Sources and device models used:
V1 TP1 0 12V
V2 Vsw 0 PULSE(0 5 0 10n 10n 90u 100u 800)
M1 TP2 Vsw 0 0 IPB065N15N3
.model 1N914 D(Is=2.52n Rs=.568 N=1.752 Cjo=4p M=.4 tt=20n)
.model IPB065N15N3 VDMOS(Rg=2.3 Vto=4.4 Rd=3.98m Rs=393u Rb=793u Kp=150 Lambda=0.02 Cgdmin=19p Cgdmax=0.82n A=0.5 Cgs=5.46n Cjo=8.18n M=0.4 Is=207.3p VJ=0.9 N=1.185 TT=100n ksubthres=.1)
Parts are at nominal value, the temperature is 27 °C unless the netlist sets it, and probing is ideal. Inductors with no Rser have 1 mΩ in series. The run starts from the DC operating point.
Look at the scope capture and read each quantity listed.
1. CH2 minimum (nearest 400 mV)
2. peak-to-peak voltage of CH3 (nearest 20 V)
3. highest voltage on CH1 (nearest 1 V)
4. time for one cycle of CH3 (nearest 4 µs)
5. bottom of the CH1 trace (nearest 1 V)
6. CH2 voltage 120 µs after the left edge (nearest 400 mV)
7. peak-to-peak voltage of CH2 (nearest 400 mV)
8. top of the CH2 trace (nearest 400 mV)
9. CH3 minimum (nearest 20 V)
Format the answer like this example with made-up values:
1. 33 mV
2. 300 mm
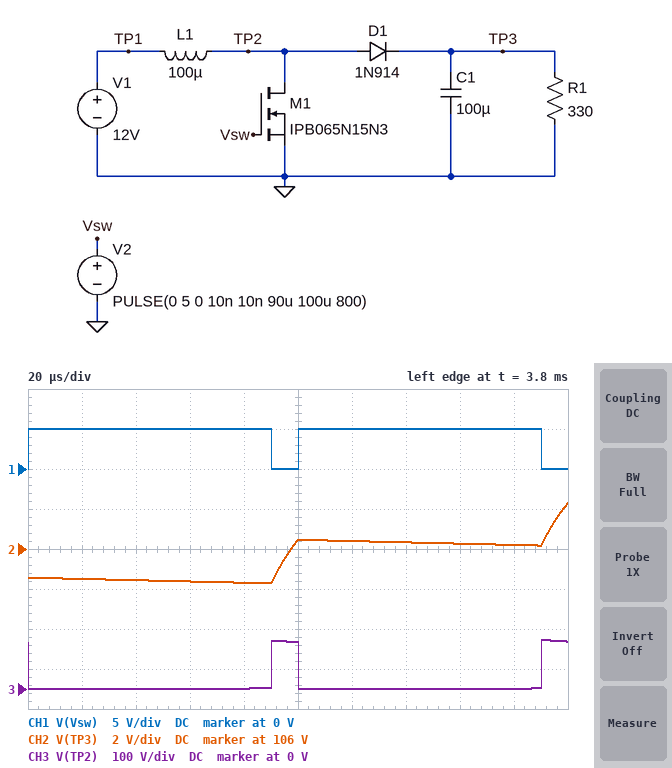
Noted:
1. 104.4 V
2. 120 V
3. 5 V
4. 100 µs
5. 0 V
6. 106.4 V
7. 4.0 V
8. 108.4 V
9. 0 V
